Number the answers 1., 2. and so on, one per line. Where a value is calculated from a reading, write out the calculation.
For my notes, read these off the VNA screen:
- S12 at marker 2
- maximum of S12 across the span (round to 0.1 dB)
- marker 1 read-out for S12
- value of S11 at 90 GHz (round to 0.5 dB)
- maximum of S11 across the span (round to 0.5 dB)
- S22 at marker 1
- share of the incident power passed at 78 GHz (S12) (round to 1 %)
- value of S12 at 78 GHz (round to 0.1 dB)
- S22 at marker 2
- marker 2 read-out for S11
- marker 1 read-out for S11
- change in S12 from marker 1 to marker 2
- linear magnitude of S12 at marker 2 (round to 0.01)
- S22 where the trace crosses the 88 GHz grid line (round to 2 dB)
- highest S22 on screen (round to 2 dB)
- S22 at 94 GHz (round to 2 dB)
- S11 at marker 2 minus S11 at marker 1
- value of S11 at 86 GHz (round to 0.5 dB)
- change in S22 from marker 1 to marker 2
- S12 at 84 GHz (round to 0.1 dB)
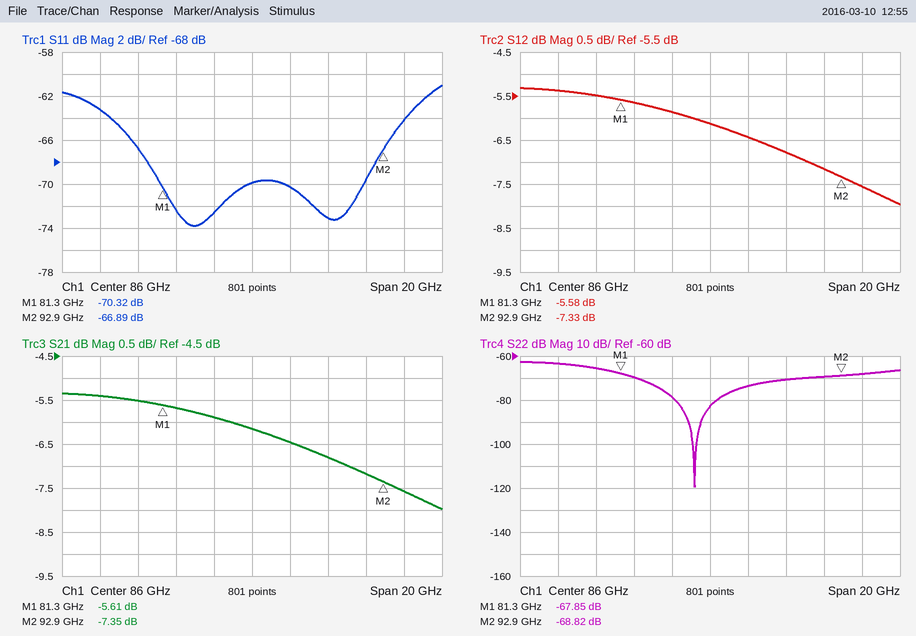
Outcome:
1. -7.33 dB
2. -5.3 dB
3. -5.58 dB
4. -73.0 dB
5. -61.0 dB
6. -67.85 dB
7. 10^(-5.4/10) ≈ 29 %
8. -5.4 dB
9. -68.82 dB
10. -66.89 dB
11. -70.32 dB
12. -7.33 − (-5.58) = -1.75 dB
13. 10^(-7.33/20) ≈ 0.43
14. -74 dB
15. -62 dB
16. -68 dB
17. -66.89 − (-70.32) = 3.43 dB
18. -70.0 dB
19. -68.82 − (-67.85) = -0.97 dB
20. -5.9 dB
